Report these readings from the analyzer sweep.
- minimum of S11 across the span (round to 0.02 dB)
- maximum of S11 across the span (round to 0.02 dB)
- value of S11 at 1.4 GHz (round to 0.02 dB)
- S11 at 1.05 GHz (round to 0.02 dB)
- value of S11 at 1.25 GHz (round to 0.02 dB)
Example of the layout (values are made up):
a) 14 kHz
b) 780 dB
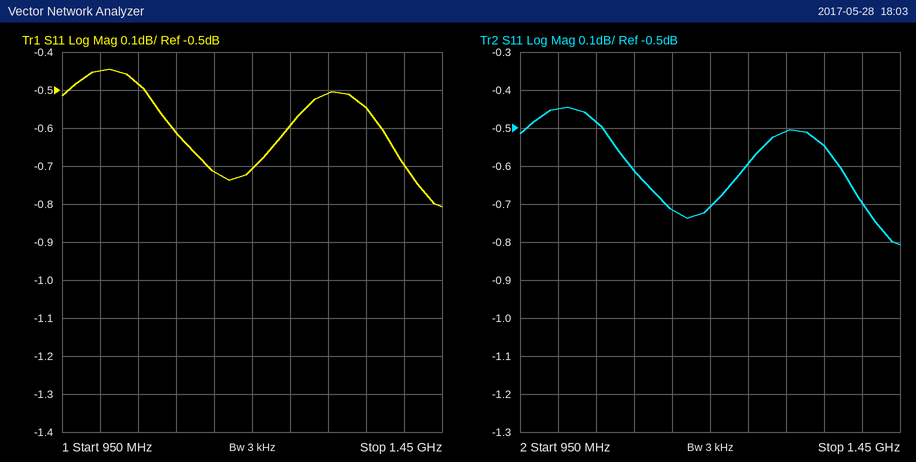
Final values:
a) -0.80 dB
b) -0.44 dB
c) -0.70 dB
d) -0.48 dB
e) -0.60 dB
